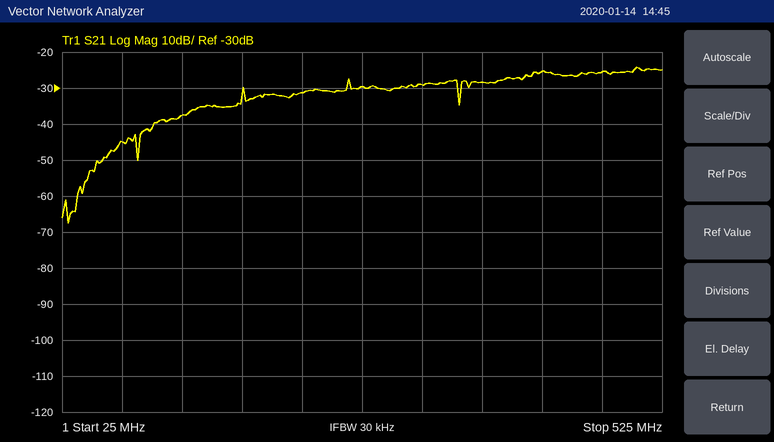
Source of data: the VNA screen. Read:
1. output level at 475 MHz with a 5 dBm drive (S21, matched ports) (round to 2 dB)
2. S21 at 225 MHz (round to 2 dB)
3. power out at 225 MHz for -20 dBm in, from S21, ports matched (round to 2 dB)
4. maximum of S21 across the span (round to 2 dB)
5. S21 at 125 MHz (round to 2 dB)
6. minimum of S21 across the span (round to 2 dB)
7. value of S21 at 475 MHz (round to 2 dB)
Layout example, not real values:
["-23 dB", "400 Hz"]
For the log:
["-20 dBm", "-32 dB", "-52 dBm", "-24 dB", "-38 dB", "-68 dB", "-26 dB"]
